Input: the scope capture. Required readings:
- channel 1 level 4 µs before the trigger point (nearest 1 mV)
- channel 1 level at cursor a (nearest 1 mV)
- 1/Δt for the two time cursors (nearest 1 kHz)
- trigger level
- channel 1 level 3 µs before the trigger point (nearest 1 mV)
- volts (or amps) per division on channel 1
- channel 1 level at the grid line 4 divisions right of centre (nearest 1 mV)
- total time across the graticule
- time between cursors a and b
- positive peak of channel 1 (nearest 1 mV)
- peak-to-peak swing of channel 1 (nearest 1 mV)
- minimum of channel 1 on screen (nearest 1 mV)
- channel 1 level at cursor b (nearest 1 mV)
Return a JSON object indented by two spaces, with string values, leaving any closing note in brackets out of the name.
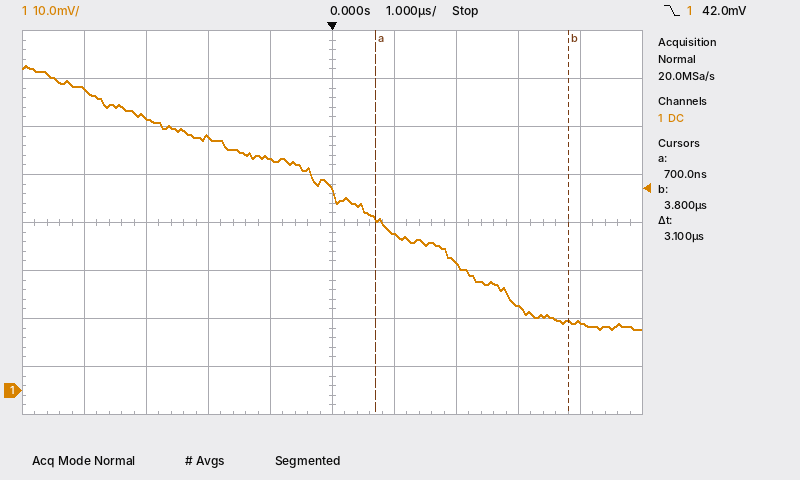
{
  "channel 1 level 4 µs before the trigger point": "63 mV",
  "channel 1 level at cursor a": "36 mV",
  "1/Δt for the two time cursors": "323 kHz",
  "trigger level": "42.0 mV",
  "channel 1 level 3 µs before the trigger point": "57 mV",
  "volts (or amps) per division on channel 1": "10 mV",
  "channel 1 level at the grid line 4 divisions right of centre": "14 mV",
  "total time across the graticule": "10 µs",
  "time between cursors a and b": "3.1 µs",
  "positive peak of channel 1": "68 mV",
  "peak-to-peak swing of channel 1": "55 mV",
  "minimum of channel 1 on screen": "13 mV",
  "channel 1 level at cursor b": "14 mV"
}
